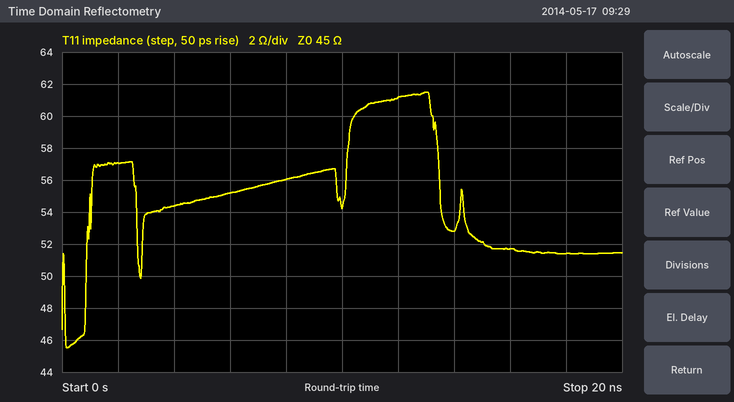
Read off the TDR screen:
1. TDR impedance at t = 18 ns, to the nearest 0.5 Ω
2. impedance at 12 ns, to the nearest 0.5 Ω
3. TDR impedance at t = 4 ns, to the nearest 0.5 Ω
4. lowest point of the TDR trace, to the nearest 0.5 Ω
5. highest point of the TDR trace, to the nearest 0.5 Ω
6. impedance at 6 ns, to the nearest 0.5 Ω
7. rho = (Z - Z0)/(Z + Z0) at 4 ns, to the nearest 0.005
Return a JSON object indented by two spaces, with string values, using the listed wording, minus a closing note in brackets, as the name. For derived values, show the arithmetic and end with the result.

{
  "TDR impedance at t = 18 ns, to the nearest 0.5 Ω": "51.5 Ω",
  "impedance at 12 ns, to the nearest 0.5 Ω": "61.0 Ω",
  "TDR impedance at t = 4 ns, to the nearest 0.5 Ω": "54.5 Ω",
  "lowest point of the TDR trace, to the nearest 0.5 Ω": "45.5 Ω",
  "highest point of the TDR trace, to the nearest 0.5 Ω": "61.5 Ω",
  "impedance at 6 ns, to the nearest 0.5 Ω": "55.0 Ω",
  "rho = (Z - Z0)/(Z + Z0) at 4 ns, to the nearest 0.005": "(54.5 − 45)/(54.5 + 45) ≈ +0.095"
}
